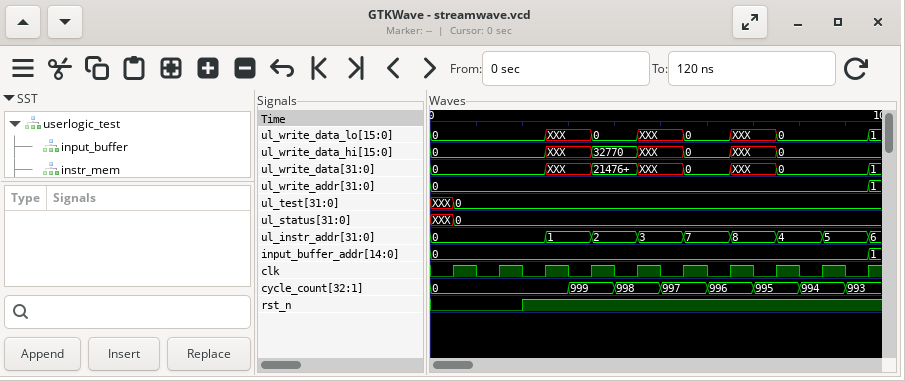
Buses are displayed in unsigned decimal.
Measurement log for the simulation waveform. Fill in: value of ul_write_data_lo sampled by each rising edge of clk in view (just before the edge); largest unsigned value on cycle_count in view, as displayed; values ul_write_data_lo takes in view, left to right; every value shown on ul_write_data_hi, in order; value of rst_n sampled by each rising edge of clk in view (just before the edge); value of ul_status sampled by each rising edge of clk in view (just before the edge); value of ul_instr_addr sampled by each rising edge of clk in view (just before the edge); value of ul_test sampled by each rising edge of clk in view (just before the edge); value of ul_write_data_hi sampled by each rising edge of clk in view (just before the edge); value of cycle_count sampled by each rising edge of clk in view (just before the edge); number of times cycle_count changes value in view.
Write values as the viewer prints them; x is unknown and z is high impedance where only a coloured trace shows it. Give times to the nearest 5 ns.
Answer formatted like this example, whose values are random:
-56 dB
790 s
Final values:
0, 0, 0, XXX, 0, XXX, 0, XXX, 0, 0
999
0, XXX, 0, XXX, 0, XXX, 0, 1
0, XXX, 32770, XXX, 0, XXX, 0
0 0 1 1 1 1 1 1 1 1
XXX, 0, 0, 0, 0, 0, 0, 0, 0, 0
0, 0, 0, 1, 2, 3, 7, 8, 4, 5
XXX, 0, 0, 0, 0, 0, 0, 0, 0, 0
0, 0, 0, XXX, 32770, XXX, 0, XXX, 0, 0
0, 0, 0, 999, 998, 997, 996, 995, 994, 993
7
